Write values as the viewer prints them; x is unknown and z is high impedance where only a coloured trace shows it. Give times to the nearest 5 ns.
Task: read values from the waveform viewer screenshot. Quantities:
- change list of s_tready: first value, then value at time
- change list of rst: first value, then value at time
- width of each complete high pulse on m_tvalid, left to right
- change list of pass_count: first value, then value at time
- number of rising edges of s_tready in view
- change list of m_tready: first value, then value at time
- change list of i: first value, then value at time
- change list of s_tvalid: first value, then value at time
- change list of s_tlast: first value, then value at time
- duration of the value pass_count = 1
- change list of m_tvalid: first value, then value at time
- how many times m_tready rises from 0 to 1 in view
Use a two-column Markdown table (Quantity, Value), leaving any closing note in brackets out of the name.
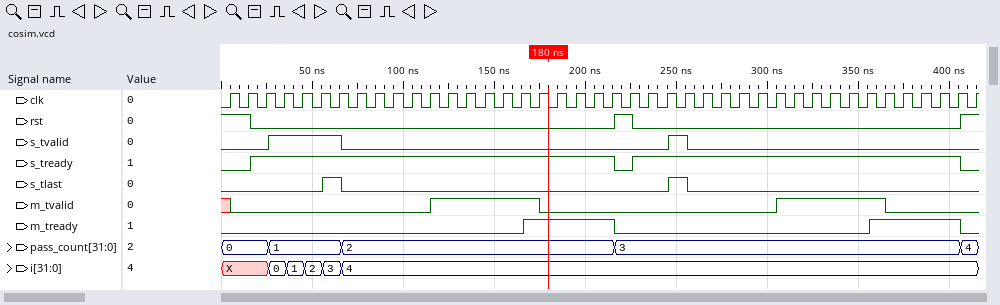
| Quantity | Value |
|---|---|
| change list of s_tready: first value, then value at time | 0, 1 at 15 ns, 0 at 215 ns, 1 at 225 ns, 0 at 405 ns |
| change list of rst: first value, then value at time | 1, 0 at 15 ns, 1 at 215 ns, 0 at 225 ns, 1 at 405 ns |
| width of each complete high pulse on m_tvalid, left to right | 60 ns, 60 ns |
| change list of pass_count: first value, then value at time | 0, 1 at 25 ns, 2 at 65 ns, 3 at 215 ns, 4 at 405 ns |
| number of rising edges of s_tready in view | 2 |
| change list of m_tready: first value, then value at time | 0, 1 at 165 ns, 0 at 215 ns, 1 at 355 ns, 0 at 405 ns |
| change list of i: first value, then value at time | X, 0 at 25 ns, 1 at 35 ns, 2 at 45 ns, 3 at 55 ns, 4 at 65 ns |
| change list of s_tvalid: first value, then value at time | 0, 1 at 25 ns, 0 at 65 ns, 1 at 245 ns, 0 at 255 ns |
| change list of s_tlast: first value, then value at time | 0, 1 at 55 ns, 0 at 65 ns, 1 at 245 ns, 0 at 255 ns |
| duration of the value pass_count = 1 | 40 ns |
| change list of m_tvalid: first value, then value at time | x, 0 at 5 ns, 1 at 115 ns, 0 at 175 ns, 1 at 305 ns, 0 at 365 ns |
| how many times m_tready rises from 0 to 1 in view | 2 |
